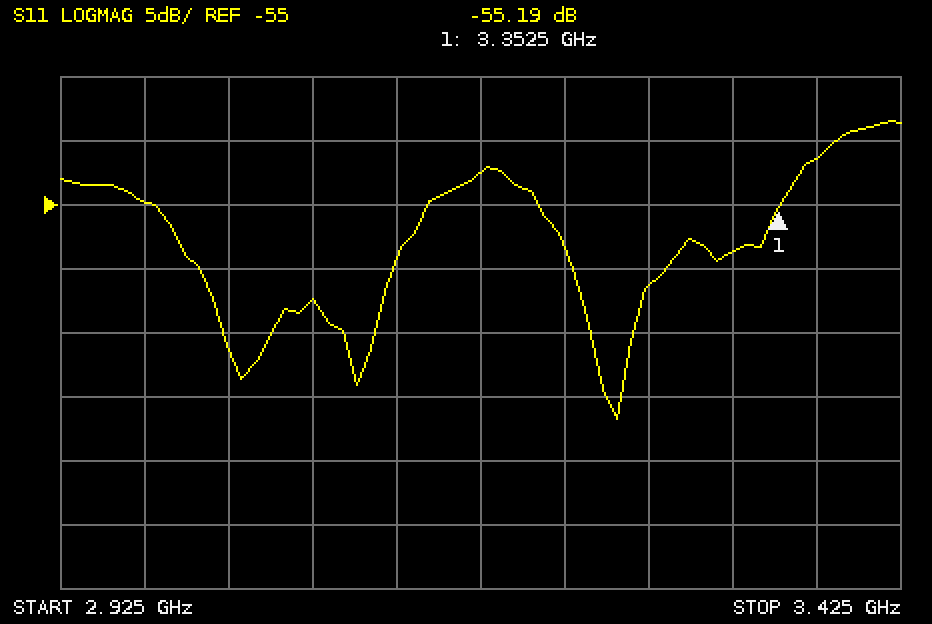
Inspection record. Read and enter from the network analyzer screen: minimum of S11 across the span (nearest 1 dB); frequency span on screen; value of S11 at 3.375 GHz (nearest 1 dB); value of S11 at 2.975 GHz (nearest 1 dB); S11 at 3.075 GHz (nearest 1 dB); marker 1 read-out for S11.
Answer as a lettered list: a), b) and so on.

a) -72 dB
b) 500 MHz
c) -51 dB
d) -55 dB
e) -62 dB
f) -55.19 dB
